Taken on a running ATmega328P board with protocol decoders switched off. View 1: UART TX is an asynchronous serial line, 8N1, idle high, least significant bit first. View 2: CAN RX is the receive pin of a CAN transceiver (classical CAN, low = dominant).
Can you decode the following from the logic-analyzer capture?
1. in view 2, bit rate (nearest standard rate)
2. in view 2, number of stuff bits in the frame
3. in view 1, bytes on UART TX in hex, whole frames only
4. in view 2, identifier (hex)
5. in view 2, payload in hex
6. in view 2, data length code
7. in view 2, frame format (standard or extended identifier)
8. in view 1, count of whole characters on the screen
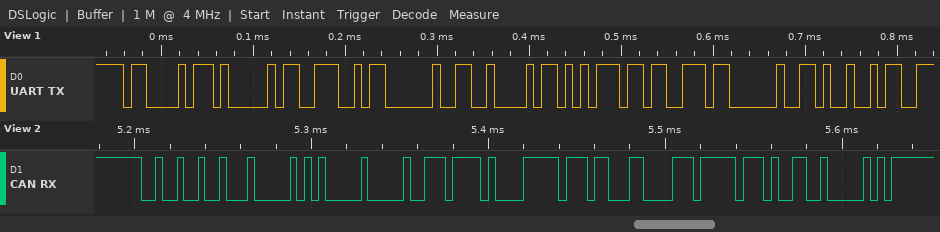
250 kbit/s
6
43 41 4E 20 42 75 73 20 49
0x249
14 00 3B D0 FF 63 0E FF
8
standard
9
